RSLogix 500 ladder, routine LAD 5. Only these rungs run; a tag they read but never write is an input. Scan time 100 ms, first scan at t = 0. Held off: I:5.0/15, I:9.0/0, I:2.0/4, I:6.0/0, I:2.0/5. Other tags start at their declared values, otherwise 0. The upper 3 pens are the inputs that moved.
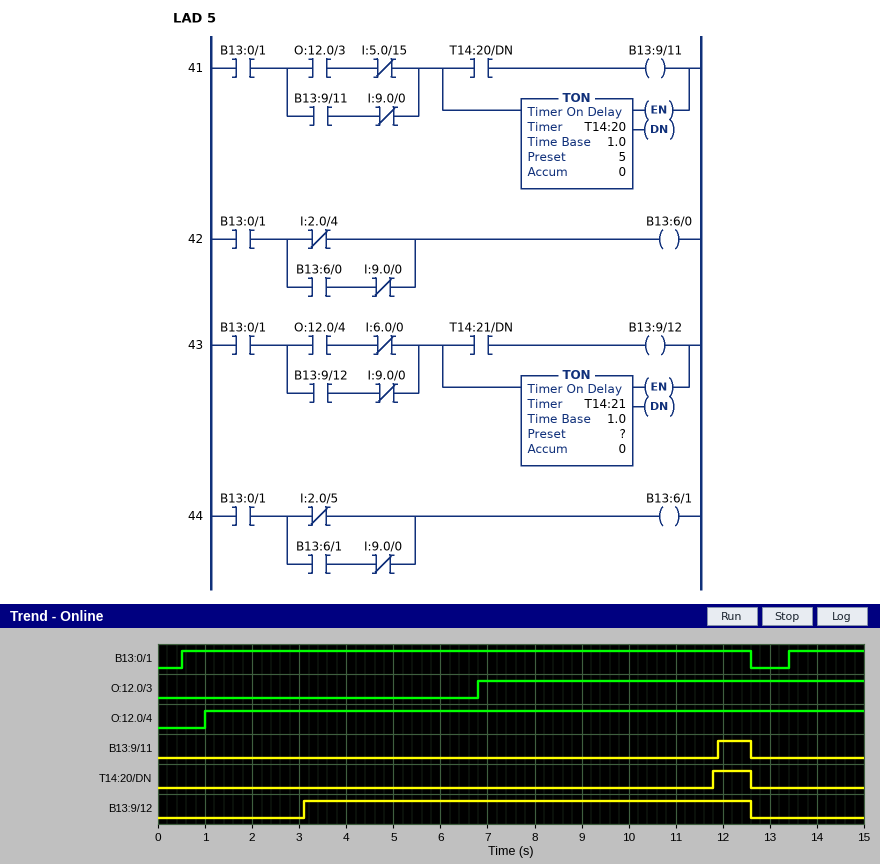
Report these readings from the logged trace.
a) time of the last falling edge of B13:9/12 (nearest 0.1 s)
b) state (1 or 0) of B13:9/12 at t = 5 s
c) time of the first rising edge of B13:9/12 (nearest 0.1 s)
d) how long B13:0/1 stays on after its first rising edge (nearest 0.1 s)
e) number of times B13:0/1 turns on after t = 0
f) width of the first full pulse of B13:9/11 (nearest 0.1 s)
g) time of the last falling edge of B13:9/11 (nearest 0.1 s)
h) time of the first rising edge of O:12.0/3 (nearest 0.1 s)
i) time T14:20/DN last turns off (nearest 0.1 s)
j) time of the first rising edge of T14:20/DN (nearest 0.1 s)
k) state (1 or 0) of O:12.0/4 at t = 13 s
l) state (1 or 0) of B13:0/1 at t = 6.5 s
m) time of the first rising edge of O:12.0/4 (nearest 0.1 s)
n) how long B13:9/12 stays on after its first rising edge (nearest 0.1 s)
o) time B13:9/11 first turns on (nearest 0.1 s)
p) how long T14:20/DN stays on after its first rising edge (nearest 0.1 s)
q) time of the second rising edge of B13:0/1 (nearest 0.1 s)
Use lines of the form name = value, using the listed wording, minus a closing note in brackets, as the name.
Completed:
time of the last falling edge of B13:9/12 = 12.6 s
state (1 or 0) of B13:9/12 at t = 5 s = 1
time of the first rising edge of B13:9/12 = 3.1 s
how long B13:0/1 stays on after its first rising edge = 12.1 s
number of times B13:0/1 turns on after t = 0 = 2
width of the first full pulse of B13:9/11 = 0.7 s
time of the last falling edge of B13:9/11 = 12.6 s
time of the first rising edge of O:12.0/3 = 6.8 s
time T14:20/DN last turns off = 12.6 s
time of the first rising edge of T14:20/DN = 11.8 s
state (1 or 0) of O:12.0/4 at t = 13 s = 1
state (1 or 0) of B13:0/1 at t = 6.5 s = 1
time of the first rising edge of O:12.0/4 = 1.0 s
how long B13:9/12 stays on after its first rising edge = 9.5 s
time B13:9/11 first turns on = 11.9 s
how long T14:20/DN stays on after its first rising edge = 0.8 s
time of the second rising edge of B13:0/1 = 13.4 s
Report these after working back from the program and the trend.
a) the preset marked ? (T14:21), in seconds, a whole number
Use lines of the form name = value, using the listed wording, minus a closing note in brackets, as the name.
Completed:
the preset marked ? (T14:21), in seconds, a whole number = 2 s
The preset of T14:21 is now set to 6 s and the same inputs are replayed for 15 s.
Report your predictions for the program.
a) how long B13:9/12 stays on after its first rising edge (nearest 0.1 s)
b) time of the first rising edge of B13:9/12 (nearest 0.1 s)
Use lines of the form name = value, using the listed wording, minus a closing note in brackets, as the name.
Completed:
how long B13:9/12 stays on after its first rising edge = 5.5 s
time of the first rising edge of B13:9/12 = 7.1 s
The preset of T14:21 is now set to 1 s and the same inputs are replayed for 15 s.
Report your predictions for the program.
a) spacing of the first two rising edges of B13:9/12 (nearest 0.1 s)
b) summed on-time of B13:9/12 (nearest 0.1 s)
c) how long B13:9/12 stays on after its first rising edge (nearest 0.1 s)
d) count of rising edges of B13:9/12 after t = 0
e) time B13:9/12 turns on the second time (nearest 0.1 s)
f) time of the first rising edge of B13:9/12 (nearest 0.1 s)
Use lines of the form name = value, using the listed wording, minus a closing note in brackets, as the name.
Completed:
spacing of the first two rising edges of B13:9/12 = 12.4 s
summed on-time of B13:9/12 = 11.0 s
how long B13:9/12 stays on after its first rising edge = 10.5 s
count of rising edges of B13:9/12 after t = 0 = 2
time B13:9/12 turns on the second time = 14.5 s
time of the first rising edge of B13:9/12 = 2.1 s
